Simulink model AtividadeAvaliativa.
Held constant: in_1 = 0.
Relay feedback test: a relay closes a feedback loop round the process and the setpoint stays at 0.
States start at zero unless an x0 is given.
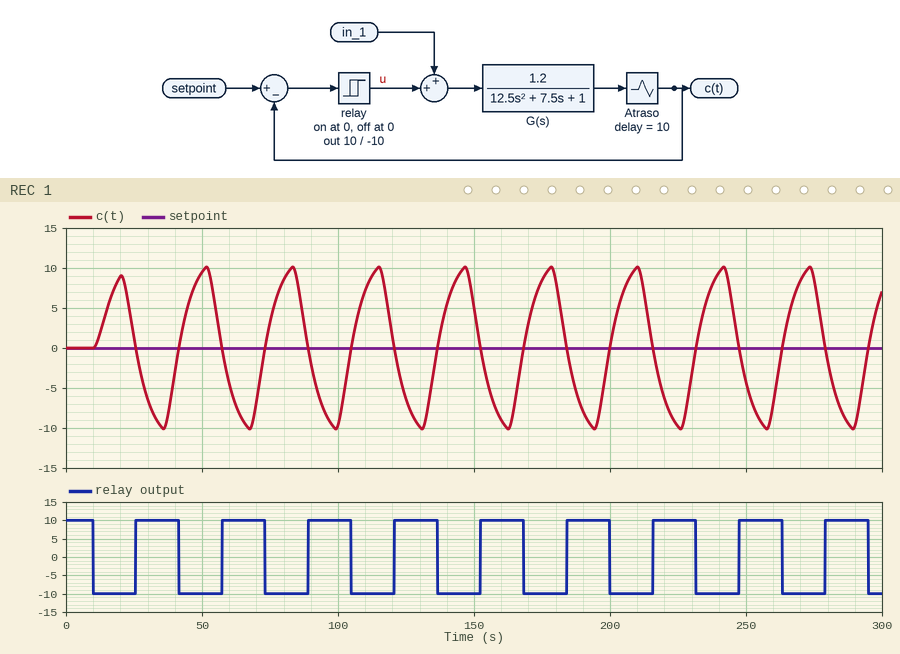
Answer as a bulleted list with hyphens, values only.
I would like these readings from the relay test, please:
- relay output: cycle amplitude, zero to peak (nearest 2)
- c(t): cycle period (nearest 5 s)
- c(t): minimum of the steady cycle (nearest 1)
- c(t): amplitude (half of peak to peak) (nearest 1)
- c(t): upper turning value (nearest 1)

- 10
- 30 s
- -10
- 10
- 10
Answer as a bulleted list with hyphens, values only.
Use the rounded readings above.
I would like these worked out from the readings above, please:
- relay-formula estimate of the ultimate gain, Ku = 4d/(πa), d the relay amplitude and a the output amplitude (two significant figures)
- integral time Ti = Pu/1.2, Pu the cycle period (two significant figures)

- 1.3
- 25 s
